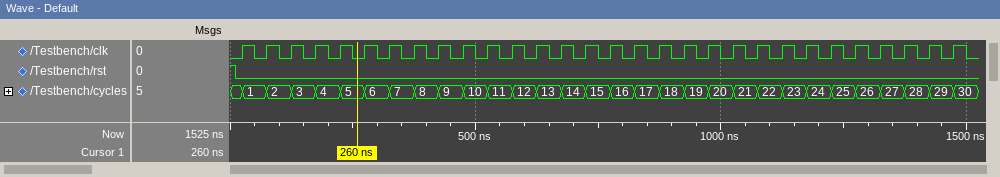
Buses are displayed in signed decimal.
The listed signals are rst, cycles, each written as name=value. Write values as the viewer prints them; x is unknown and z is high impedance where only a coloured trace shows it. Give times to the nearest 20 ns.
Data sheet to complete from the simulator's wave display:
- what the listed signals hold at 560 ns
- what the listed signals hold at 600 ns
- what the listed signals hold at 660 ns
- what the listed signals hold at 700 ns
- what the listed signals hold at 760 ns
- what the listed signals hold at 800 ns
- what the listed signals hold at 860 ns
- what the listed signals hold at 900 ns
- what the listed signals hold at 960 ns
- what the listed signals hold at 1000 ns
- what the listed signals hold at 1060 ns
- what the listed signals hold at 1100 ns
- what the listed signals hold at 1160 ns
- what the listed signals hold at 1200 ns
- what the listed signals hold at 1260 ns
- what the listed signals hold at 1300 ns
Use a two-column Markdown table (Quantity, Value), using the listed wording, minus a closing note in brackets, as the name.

| Quantity | Value |
|---|---|
| what the listed signals hold at 560 ns | rst=0, cycles=11 |
| what the listed signals hold at 600 ns | rst=0, cycles=12 |
| what the listed signals hold at 660 ns | rst=0, cycles=13 |
| what the listed signals hold at 700 ns | rst=0, cycles=14 |
| what the listed signals hold at 760 ns | rst=0, cycles=15 |
| what the listed signals hold at 800 ns | rst=0, cycles=16 |
| what the listed signals hold at 860 ns | rst=0, cycles=17 |
| what the listed signals hold at 900 ns | rst=0, cycles=18 |
| what the listed signals hold at 960 ns | rst=0, cycles=19 |
| what the listed signals hold at 1000 ns | rst=0, cycles=20 |
| what the listed signals hold at 1060 ns | rst=0, cycles=21 |
| what the listed signals hold at 1100 ns | rst=0, cycles=22 |
| what the listed signals hold at 1160 ns | rst=0, cycles=23 |
| what the listed signals hold at 1200 ns | rst=0, cycles=24 |
| what the listed signals hold at 1260 ns | rst=0, cycles=25 |
| what the listed signals hold at 1300 ns | rst=0, cycles=26 |
